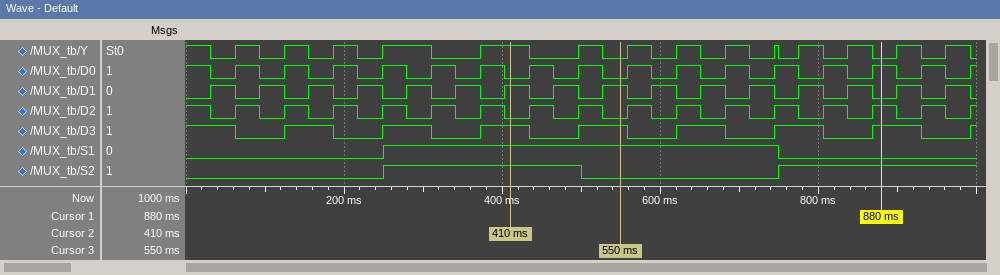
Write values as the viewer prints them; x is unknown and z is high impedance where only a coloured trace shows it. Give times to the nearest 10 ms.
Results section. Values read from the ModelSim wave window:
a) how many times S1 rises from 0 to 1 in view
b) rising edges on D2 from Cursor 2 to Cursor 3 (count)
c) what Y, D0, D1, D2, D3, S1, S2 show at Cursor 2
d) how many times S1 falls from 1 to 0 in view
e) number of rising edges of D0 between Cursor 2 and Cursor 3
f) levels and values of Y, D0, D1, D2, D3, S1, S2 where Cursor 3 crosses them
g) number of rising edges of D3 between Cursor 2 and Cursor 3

1
2
Y=1, D0=0, D1=1, D2=0, D3=1, S1=1, S2=1
1
2
Y=0, D0=0, D1=1, D2=0, D3=1, S1=1, S2=0
1
